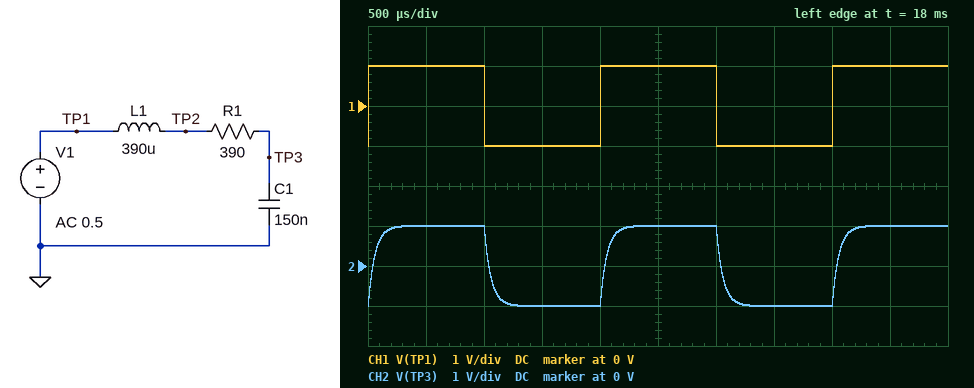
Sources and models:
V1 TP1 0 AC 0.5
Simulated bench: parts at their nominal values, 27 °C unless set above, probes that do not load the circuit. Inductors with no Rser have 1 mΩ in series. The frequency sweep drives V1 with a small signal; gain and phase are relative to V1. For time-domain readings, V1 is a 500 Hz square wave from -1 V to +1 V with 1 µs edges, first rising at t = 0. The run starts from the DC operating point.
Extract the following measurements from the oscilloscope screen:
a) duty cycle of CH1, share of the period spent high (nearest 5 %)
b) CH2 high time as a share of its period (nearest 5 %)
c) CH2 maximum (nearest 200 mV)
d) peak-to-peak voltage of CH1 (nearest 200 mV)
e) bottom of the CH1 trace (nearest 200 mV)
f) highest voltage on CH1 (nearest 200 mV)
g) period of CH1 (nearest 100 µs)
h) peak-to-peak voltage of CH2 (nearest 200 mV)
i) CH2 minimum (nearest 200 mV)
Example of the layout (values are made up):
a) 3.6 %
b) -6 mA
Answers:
a) 50 %
b) 50 %
c) 1.0 V
d) 2.0 V
e) -1.0 V
f) 1.0 V
g) 2.0 ms
h) 2.0 V
i) -1.0 V
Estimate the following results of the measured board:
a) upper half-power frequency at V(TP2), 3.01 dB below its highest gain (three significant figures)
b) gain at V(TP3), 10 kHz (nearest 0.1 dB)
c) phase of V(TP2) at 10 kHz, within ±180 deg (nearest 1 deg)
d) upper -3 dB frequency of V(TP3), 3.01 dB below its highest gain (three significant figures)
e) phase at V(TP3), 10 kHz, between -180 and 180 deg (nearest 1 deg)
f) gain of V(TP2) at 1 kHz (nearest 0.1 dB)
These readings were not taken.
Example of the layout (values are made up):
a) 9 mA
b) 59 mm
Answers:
a) 157 kHz
b) -11.5 dB
c) -3 deg
d) 2.77 kHz
e) -78 deg
f) 0 dB
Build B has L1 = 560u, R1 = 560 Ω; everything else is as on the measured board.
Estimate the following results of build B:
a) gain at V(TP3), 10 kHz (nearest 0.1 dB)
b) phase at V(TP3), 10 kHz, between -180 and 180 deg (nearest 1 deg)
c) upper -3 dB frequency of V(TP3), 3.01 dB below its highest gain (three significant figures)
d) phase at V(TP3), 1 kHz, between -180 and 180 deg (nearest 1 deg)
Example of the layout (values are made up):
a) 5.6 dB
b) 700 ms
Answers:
a) -14.5 dB
b) -83 deg
c) 1.92 kHz
d) -28 deg
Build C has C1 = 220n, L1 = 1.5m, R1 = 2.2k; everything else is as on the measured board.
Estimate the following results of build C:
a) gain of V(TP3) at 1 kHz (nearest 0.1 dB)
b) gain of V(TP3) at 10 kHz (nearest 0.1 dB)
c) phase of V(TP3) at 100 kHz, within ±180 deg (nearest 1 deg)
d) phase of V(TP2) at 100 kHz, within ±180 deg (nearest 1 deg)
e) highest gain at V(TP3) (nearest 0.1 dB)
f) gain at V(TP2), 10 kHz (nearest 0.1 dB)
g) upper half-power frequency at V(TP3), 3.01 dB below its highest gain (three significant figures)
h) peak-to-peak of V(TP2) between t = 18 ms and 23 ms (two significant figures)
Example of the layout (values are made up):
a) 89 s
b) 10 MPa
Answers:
a) -10.1 dB
b) -29.7 dB
c) -113 deg
d) -23 deg
e) 0 dB
f) 0 dB
g) 329 Hz
h) 2.0 V
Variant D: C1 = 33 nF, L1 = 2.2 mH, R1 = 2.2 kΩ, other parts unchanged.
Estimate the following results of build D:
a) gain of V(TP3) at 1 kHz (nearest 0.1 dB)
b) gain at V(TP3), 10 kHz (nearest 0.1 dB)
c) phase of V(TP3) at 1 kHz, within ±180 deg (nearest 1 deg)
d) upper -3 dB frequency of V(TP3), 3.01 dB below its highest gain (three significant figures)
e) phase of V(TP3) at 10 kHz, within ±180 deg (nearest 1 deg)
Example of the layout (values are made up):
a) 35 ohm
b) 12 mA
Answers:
a) -0.8 dB
b) -13.3 dB
c) -25 deg
d) 2.22 kHz
e) -81 deg
